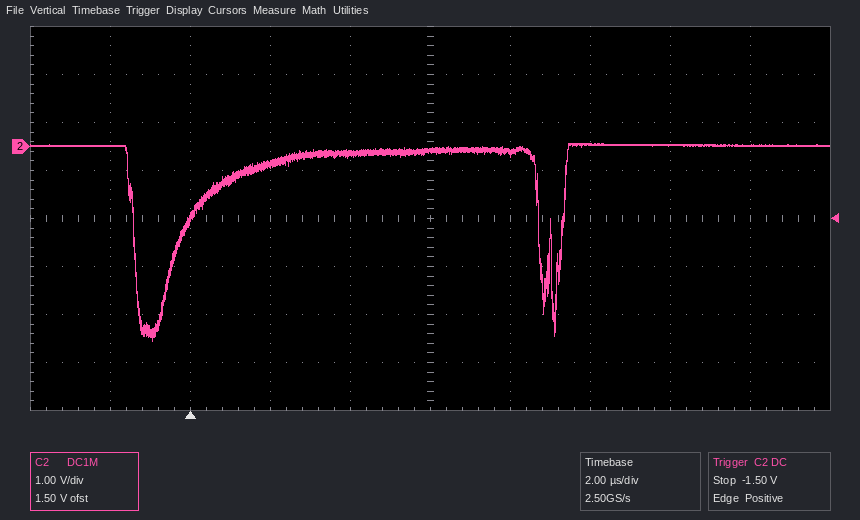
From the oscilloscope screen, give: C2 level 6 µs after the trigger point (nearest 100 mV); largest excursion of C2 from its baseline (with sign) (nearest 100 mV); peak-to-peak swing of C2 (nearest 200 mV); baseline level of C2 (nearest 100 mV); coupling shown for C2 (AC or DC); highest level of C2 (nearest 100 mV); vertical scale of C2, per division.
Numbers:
-100 mV
-4.1 V
4.2 V
0.0 V
DC
100 mV
1 V
